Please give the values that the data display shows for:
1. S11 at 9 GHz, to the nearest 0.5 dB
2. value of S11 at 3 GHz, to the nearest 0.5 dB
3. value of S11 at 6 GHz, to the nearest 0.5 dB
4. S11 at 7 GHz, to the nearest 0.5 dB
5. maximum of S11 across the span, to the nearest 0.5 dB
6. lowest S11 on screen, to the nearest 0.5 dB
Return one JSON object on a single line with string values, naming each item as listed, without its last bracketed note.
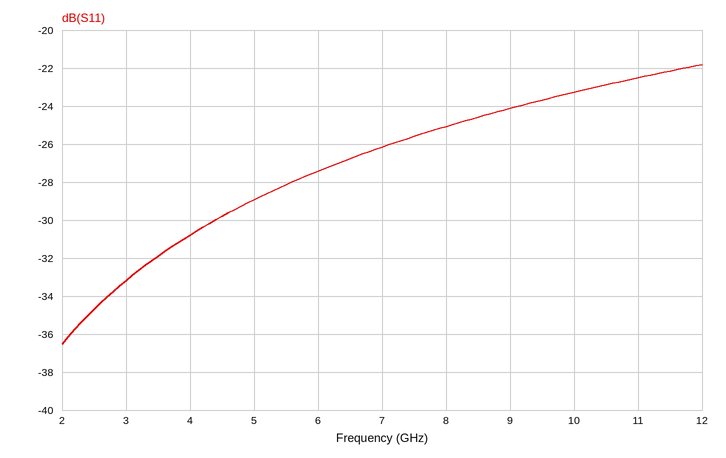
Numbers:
{"S11 at 9 GHz, to the nearest 0.5 dB": "-24.0 dB", "value of S11 at 3 GHz, to the nearest 0.5 dB": "-33.0 dB", "value of S11 at 6 GHz, to the nearest 0.5 dB": "-27.5 dB", "S11 at 7 GHz, to the nearest 0.5 dB": "-26.0 dB", "maximum of S11 across the span, to the nearest 0.5 dB": "-22.0 dB", "lowest S11 on screen, to the nearest 0.5 dB": "-36.5 dB"}
